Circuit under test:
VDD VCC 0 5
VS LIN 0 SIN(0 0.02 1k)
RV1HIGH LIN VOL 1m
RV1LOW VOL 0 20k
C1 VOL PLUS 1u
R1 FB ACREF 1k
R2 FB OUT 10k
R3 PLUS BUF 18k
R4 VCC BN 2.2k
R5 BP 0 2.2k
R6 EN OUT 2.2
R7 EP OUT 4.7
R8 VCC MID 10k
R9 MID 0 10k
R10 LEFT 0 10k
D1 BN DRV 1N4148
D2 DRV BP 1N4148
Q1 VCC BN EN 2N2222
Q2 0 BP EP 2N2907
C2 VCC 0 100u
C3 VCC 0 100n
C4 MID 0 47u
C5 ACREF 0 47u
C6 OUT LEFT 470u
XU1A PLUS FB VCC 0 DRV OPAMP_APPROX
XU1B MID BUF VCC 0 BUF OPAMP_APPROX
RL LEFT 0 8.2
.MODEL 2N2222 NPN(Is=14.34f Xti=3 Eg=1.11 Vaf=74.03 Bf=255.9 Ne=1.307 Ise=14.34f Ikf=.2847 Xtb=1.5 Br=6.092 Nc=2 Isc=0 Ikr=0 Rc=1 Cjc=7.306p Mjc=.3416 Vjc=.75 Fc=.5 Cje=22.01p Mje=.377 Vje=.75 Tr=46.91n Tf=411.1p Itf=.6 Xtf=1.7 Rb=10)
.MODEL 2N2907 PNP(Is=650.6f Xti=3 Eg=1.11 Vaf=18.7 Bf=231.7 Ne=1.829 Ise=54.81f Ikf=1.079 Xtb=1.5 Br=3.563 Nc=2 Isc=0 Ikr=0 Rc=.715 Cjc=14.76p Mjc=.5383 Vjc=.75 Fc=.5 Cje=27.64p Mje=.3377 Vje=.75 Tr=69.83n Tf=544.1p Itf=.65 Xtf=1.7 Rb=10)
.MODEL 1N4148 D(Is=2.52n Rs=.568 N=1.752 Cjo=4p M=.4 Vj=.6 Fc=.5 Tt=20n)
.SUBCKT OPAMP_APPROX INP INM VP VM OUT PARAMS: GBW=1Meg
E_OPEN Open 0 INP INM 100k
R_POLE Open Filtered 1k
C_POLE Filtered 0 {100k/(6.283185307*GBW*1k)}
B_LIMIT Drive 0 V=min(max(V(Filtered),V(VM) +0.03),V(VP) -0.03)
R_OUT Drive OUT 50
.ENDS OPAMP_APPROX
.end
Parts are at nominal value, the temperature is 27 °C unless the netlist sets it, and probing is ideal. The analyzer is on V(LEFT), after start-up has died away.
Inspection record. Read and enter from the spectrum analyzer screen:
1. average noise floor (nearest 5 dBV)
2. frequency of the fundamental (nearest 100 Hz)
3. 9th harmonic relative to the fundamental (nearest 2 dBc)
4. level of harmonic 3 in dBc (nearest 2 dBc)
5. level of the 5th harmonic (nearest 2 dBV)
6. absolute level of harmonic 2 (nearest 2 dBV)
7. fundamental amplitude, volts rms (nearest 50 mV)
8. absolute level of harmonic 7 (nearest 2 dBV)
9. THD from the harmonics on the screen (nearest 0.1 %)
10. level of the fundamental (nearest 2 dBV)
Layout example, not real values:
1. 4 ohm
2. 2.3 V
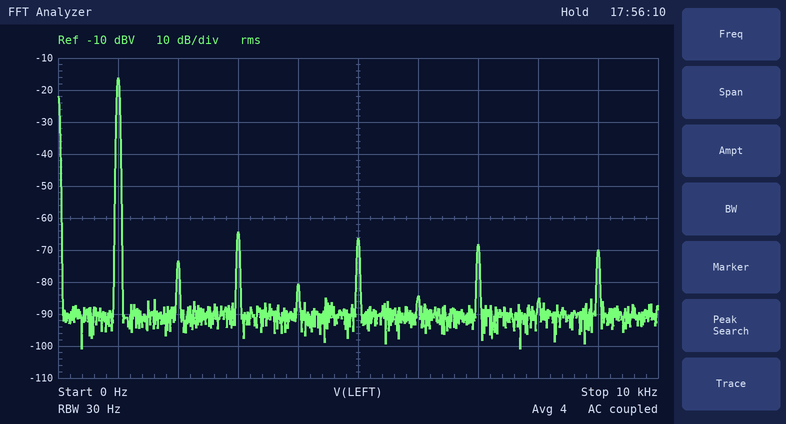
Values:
1. -90 dBV
2. 1.0 kHz
3. -54 dBc
4. -48 dBc
5. -66 dBV
6. -74 dBV
7. 150 mV
8. -68 dBV
9. 0.6 %
10. -16 dBV
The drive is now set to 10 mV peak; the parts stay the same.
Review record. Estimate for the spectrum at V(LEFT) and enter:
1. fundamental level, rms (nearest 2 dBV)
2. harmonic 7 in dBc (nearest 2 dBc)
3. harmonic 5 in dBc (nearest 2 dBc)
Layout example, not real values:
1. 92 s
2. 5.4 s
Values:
1. -22 dBV
2. -50 dBc
3. -48 dBc
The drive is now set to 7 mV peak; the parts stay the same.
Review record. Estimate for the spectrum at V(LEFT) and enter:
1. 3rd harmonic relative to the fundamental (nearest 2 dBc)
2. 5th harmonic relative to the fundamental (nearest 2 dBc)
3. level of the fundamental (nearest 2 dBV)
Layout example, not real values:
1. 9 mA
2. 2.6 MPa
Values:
1. -44 dBc
2. -48 dBc
3. -26 dBV
